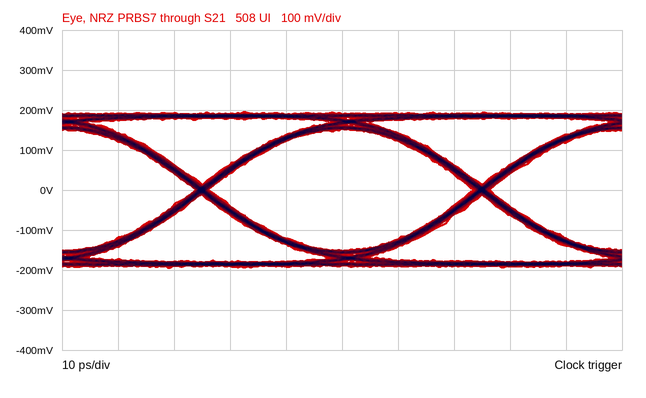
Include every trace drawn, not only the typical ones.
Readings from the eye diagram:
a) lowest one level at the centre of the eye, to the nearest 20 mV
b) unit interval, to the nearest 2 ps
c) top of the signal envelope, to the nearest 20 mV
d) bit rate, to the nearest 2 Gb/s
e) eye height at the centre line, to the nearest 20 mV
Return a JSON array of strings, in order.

["160 mV", "50 ps", "200 mV", "20 Gb/s", "300 mV"]
